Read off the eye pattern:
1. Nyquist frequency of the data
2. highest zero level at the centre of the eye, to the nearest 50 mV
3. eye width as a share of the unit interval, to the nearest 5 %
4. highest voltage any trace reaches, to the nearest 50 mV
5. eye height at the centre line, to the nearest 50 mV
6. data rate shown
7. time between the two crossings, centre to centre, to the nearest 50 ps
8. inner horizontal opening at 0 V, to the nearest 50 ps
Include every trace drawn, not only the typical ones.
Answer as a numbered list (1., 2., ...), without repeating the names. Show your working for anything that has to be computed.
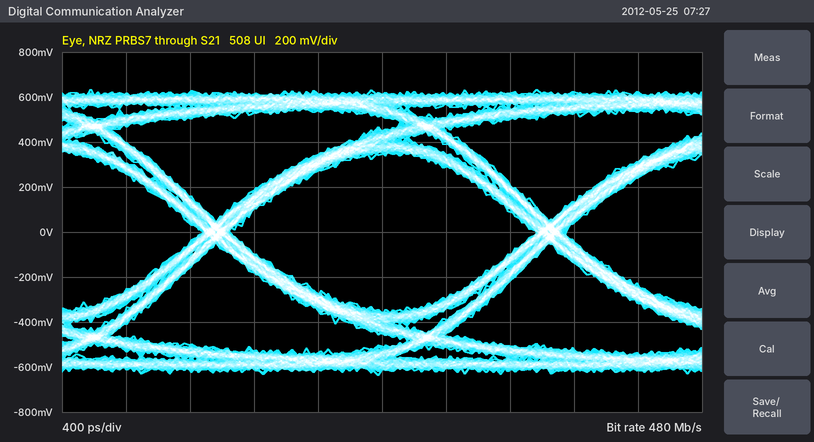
1. 240 MHz
2. -350 mV
3. 1.90 ns / 2.10 ns ≈ 90 %
4. 650 mV
5. 700 mV
6. 480 Mb/s
7. 2.10 ns
8. 1.90 ns
